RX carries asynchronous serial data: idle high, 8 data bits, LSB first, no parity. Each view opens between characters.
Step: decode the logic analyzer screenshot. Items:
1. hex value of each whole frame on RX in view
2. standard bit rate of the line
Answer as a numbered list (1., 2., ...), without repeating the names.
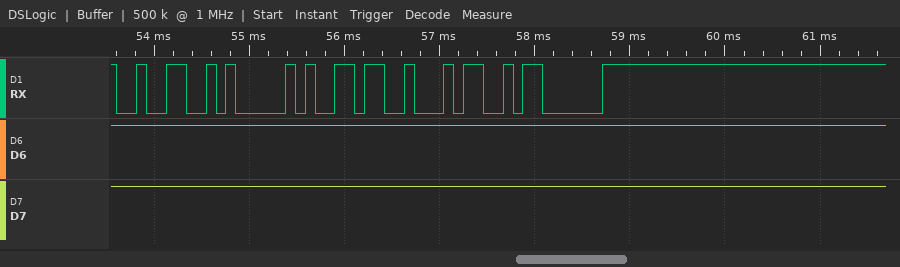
1. 32, 41, 36, 34, 03
2. 9600 baud
